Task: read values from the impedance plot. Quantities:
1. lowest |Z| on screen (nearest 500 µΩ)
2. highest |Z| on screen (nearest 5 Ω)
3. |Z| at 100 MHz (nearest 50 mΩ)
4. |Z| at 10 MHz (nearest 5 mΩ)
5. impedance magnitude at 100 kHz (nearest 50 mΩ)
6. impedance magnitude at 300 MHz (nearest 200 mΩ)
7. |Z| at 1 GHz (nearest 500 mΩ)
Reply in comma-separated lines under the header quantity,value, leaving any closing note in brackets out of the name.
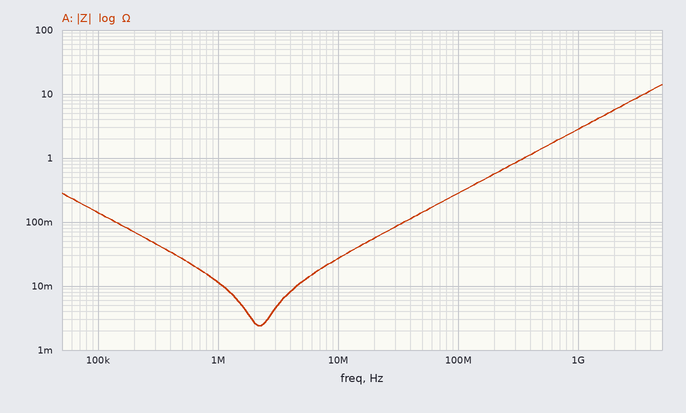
quantity,value
lowest |Z| on screen,2.5 mΩ
highest |Z| on screen,15 Ω
|Z| at 100 MHz,300 mΩ
|Z| at 10 MHz,25 mΩ
impedance magnitude at 100 kHz,150 mΩ
impedance magnitude at 300 MHz,800 mΩ
|Z| at 1 GHz,3.0 Ω
